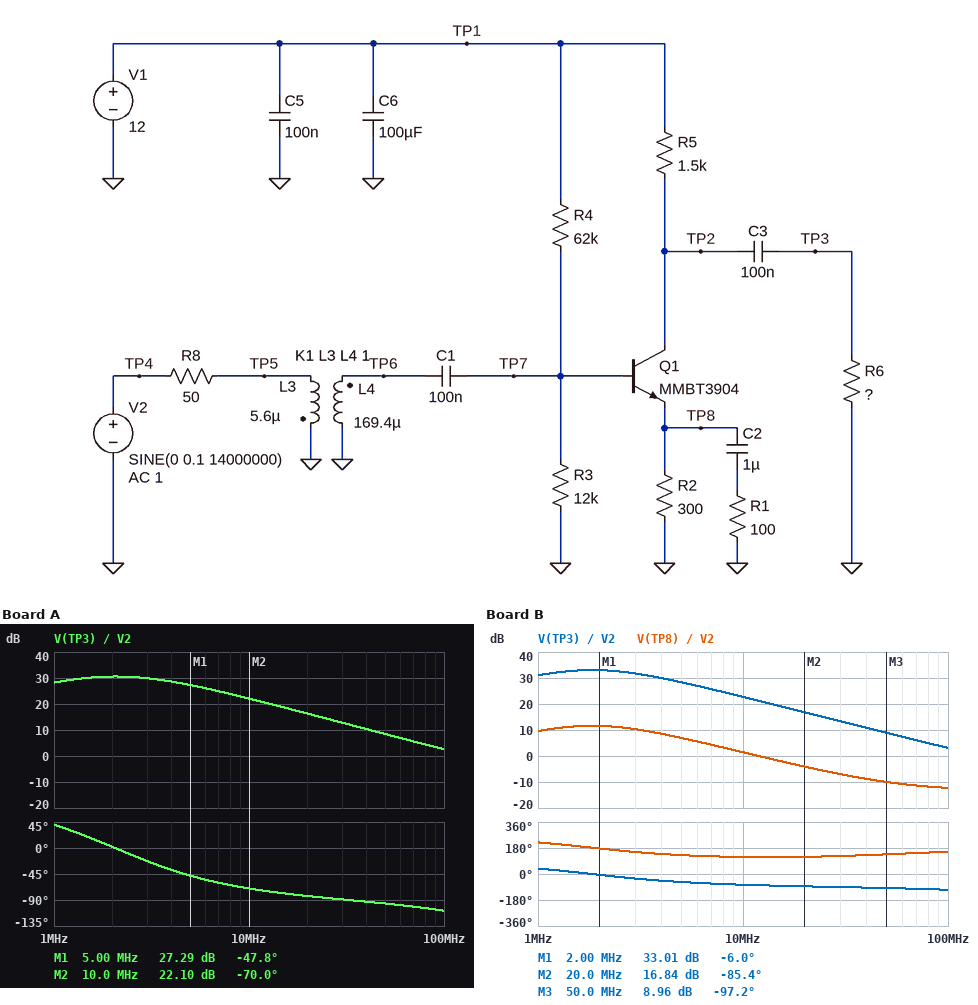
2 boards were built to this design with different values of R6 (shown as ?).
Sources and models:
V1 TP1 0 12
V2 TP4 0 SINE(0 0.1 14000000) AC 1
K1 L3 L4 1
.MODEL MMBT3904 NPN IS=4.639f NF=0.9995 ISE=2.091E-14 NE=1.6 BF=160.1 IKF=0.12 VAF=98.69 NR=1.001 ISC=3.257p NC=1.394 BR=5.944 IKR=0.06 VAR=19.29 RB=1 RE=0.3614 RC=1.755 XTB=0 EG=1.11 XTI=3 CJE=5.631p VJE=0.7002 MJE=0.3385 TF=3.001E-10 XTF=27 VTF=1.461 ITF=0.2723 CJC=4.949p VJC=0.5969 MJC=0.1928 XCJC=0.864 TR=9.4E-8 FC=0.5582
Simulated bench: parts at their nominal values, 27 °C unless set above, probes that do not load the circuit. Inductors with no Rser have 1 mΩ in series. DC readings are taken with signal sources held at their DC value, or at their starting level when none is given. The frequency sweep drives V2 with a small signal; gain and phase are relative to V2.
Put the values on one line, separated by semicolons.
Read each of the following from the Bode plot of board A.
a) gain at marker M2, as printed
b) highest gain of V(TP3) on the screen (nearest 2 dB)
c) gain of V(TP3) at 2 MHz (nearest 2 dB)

22.10 dB; 30 dB; 30 dB
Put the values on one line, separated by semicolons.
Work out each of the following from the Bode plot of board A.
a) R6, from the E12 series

1.2 kΩ
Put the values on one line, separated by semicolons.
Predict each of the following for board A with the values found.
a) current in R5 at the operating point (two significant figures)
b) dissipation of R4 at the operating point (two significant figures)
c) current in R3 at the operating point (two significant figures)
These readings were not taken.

3.4 mA; 1.7 mW; 140 µA
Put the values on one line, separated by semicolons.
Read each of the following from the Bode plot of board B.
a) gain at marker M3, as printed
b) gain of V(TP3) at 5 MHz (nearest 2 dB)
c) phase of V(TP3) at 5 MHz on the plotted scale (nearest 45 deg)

8.96 dB; 28 dB; -45 deg
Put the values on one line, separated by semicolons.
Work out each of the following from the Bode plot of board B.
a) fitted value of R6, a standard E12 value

2.2 kΩ
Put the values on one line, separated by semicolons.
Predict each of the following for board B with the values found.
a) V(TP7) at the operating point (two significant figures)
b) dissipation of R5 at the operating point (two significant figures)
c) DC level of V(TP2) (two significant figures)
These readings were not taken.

1.7 V; 17 mW; 6.9 V
